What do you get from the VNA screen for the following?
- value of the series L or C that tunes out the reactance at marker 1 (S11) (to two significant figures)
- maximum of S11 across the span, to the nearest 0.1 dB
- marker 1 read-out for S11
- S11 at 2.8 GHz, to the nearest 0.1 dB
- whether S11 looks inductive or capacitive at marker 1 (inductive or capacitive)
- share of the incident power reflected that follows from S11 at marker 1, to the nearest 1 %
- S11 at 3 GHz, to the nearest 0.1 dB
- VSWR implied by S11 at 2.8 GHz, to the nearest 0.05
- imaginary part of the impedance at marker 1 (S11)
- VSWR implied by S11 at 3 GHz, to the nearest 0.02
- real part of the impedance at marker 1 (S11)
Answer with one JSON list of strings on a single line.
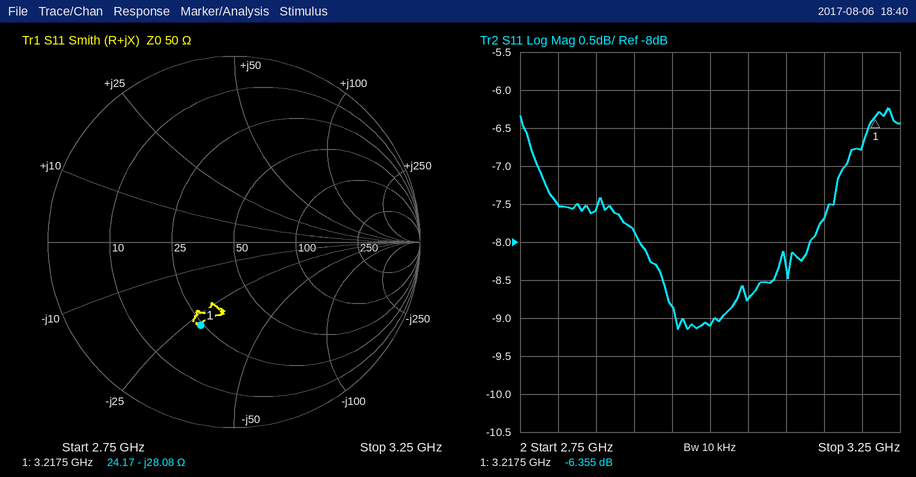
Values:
["1.4 nH", "-6.2 dB", "-6.355 dB", "-7.5 dB", "capacitive", "23 %", "-9.1 dB", "2.45", "-28.08 Ω", "2.08", "24.17 Ω"]
